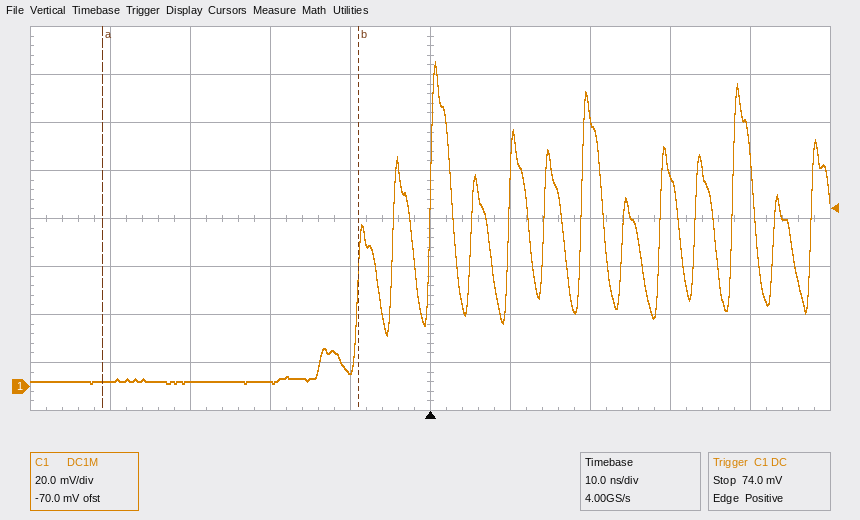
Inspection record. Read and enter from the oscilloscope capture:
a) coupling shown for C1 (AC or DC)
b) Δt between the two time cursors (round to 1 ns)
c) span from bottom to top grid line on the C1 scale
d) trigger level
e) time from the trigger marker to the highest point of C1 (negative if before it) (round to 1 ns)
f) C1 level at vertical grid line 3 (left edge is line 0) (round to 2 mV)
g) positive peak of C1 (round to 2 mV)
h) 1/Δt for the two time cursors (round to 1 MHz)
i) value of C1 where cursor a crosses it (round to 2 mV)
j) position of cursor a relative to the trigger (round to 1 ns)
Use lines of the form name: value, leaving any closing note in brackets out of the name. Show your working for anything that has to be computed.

coupling shown for C1: DC
Δt between the two time cursors: 32 ns
span from bottom to top grid line on the C1 scale: 160 mV
trigger level: 74.0 mV
time from the trigger marker to the highest point of C1 (negative if before it): +1 ns
C1 level at vertical grid line 3 (left edge is line 0): 2 mV
positive peak of C1: 136 mV
1/Δt for the two time cursors: 1 / 32 ns ≈ 31 MHz
value of C1 where cursor a crosses it: 2 mV
position of cursor a relative to the trigger: -41 ns
